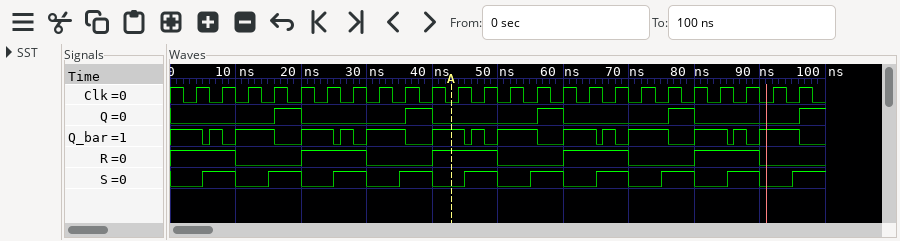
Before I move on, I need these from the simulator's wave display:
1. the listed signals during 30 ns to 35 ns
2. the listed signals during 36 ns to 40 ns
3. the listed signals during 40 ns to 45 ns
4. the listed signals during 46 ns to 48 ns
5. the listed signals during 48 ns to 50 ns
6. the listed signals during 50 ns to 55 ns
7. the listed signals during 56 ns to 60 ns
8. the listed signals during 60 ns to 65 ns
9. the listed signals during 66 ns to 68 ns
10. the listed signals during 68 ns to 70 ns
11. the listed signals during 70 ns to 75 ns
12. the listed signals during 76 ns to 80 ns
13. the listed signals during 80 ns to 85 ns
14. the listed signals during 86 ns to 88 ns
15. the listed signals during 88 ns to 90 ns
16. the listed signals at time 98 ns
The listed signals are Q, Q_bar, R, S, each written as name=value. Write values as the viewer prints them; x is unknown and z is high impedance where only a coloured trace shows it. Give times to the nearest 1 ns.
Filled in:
Q=0, Q_bar=1, R=0, S=0
Q=1, Q_bar=0, R=0, S=1
Q=0, Q_bar=1, R=1, S=0
Q=0, Q_bar=1, R=1, S=1
Q=0, Q_bar=0, R=1, S=1
Q=0, Q_bar=1, R=0, S=0
Q=1, Q_bar=0, R=0, S=1
Q=0, Q_bar=1, R=1, S=0
Q=0, Q_bar=1, R=1, S=1
Q=0, Q_bar=0, R=1, S=1
Q=0, Q_bar=1, R=0, S=0
Q=1, Q_bar=0, R=0, S=1
Q=0, Q_bar=1, R=1, S=0
Q=0, Q_bar=1, R=1, S=1
Q=0, Q_bar=0, R=1, S=1
Q=1, Q_bar=0, R=0, S=1
